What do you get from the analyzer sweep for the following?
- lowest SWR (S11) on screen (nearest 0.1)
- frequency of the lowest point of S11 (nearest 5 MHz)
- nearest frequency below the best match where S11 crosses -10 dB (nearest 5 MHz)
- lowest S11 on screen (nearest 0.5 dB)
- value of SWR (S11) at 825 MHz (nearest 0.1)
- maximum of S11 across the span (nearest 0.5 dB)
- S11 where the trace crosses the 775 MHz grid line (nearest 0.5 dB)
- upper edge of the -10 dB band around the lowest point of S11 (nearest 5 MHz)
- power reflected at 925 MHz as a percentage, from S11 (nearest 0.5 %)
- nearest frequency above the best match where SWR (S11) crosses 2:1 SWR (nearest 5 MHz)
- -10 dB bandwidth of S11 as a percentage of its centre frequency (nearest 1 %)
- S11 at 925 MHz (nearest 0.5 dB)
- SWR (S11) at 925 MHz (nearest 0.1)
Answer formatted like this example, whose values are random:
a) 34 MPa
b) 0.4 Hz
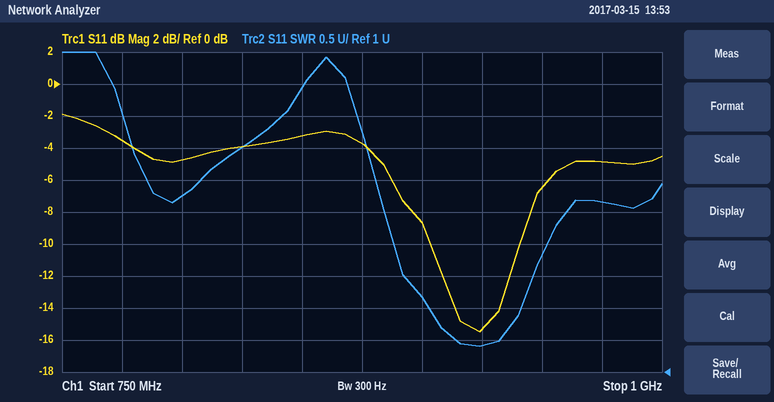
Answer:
a) 1.4
b) 925 MHz
c) 905 MHz
d) -15.5 dB
e) 4.5
f) -2.0 dB
g) -3.5 dB
h) 940 MHz
i) 3.0 %
j) 940 MHz
k) 4 %
l) -15.5 dB
m) 1.4
